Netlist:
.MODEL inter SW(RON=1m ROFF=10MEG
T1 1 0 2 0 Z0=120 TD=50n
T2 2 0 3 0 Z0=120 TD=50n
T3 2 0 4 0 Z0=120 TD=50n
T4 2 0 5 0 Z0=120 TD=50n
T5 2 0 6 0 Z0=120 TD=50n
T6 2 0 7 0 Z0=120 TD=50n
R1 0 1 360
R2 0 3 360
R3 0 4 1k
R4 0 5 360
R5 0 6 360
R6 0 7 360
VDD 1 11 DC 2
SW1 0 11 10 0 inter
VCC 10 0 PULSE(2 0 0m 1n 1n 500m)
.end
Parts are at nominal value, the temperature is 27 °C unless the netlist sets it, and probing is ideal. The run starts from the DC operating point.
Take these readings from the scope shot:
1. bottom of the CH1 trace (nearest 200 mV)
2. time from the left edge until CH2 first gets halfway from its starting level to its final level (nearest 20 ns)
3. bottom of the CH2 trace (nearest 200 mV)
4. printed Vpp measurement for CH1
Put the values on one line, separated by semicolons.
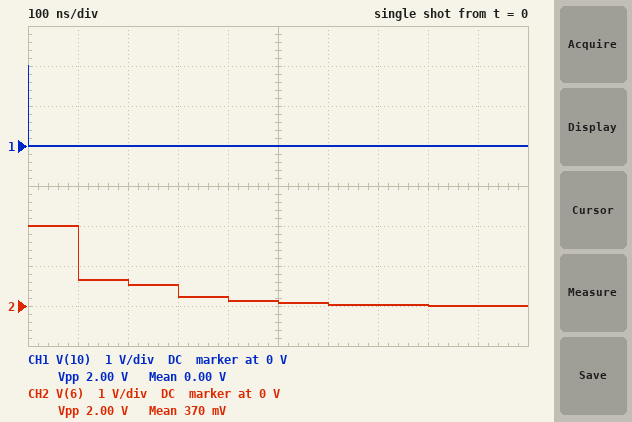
0 V; 100 ns; 0 V; 2.00 V
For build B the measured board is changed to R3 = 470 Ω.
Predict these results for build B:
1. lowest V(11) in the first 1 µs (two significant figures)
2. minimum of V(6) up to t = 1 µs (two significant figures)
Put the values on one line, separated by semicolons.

-2.9 V; 3.5 mV
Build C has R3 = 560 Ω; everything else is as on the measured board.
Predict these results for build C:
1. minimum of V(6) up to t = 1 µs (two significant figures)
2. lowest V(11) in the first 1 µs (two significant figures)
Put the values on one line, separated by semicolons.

4.8 mV; -2.8 V
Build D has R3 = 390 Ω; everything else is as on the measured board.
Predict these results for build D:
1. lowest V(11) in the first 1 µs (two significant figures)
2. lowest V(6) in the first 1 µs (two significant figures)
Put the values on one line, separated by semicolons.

-3.0 V; 2.4 mV
